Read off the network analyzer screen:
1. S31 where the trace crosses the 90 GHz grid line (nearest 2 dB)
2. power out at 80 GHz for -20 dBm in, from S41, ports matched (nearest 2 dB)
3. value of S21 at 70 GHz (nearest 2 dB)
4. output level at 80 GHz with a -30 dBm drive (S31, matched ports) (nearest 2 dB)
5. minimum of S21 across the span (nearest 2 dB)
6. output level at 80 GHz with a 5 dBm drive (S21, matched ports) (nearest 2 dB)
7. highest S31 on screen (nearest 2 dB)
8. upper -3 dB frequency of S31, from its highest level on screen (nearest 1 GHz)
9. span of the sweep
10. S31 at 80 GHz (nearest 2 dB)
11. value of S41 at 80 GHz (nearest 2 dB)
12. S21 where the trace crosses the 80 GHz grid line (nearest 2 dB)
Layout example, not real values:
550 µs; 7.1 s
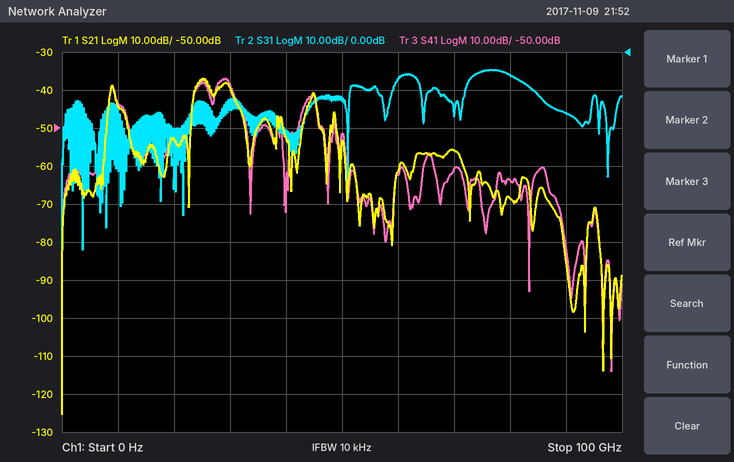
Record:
-16 dB; -84 dBm; -56 dB; -36 dBm; -126 dB; -64 dBm; -4 dB; 82 GHz; 100 GHz; -6 dB; -64 dB; -68 dB
